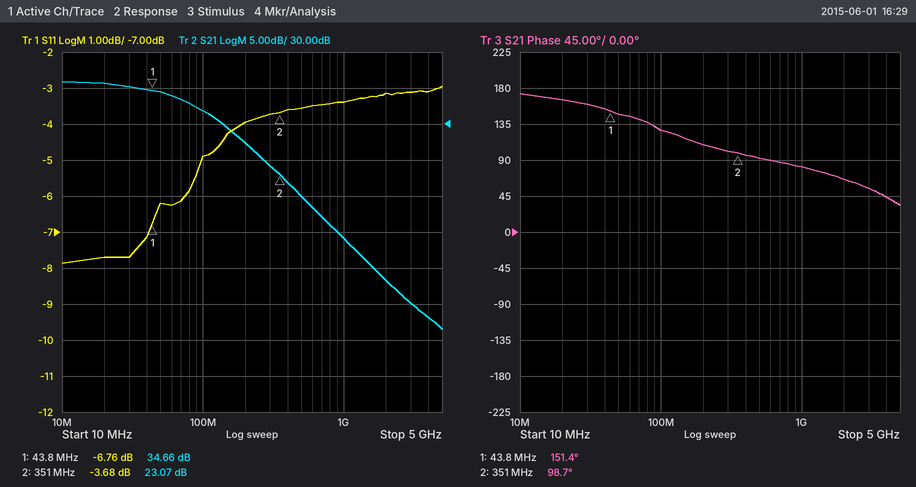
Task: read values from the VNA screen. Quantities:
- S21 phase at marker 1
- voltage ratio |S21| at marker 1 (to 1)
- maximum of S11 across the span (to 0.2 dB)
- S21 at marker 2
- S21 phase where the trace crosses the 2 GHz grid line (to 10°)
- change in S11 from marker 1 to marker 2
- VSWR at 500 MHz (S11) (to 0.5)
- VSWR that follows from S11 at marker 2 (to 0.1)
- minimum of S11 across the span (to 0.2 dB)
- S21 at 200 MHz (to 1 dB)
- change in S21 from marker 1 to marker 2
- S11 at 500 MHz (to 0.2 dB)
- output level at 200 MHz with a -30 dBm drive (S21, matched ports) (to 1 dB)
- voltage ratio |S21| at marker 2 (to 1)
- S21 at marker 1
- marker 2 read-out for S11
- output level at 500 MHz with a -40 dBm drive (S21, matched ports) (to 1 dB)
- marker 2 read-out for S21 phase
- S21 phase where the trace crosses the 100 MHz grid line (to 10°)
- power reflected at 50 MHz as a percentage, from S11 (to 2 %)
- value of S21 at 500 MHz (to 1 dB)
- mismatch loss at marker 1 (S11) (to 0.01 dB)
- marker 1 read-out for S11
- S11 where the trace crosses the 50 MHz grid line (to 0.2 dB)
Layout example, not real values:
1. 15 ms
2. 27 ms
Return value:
1. 151.4°
2. 54
3. -3.0 dB
4. 23.07 dB
5. 70°
6. 3.08 dB
7. 5.0
8. 4.8
9. -7.8 dB
10. 27 dB
11. -11.59 dB
12. -3.6 dB
13. -3 dBm
14. 14
15. 34.66 dB
16. -3.68 dB
17. -20 dBm
18. 98.7°
19. 130°
20. 24 %
21. 20 dB
22. 1.03 dB
23. -6.76 dB
24. -6.2 dB
